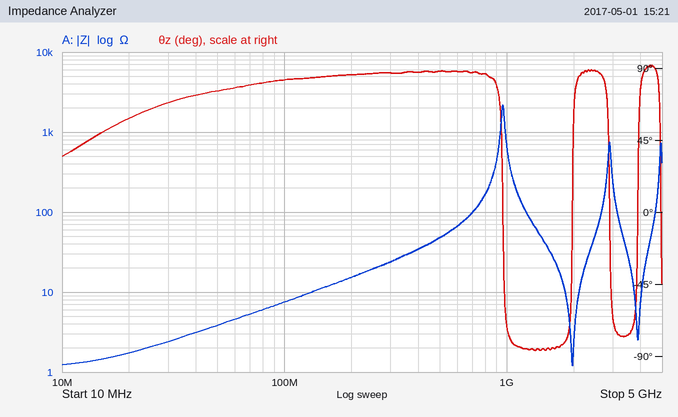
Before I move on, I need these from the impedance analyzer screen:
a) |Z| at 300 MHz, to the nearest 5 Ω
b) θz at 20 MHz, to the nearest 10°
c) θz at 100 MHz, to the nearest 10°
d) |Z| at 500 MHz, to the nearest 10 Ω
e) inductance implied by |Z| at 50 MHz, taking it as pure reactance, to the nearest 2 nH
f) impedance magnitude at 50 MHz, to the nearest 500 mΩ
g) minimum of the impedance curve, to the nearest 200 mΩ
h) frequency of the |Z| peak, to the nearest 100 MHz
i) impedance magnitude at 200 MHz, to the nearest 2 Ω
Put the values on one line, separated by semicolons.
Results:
25 Ω; 60°; 80°; 50 Ω; 12 nH; 4.0 Ω; 1.2 Ω; 1.0 GHz; 16 Ω
